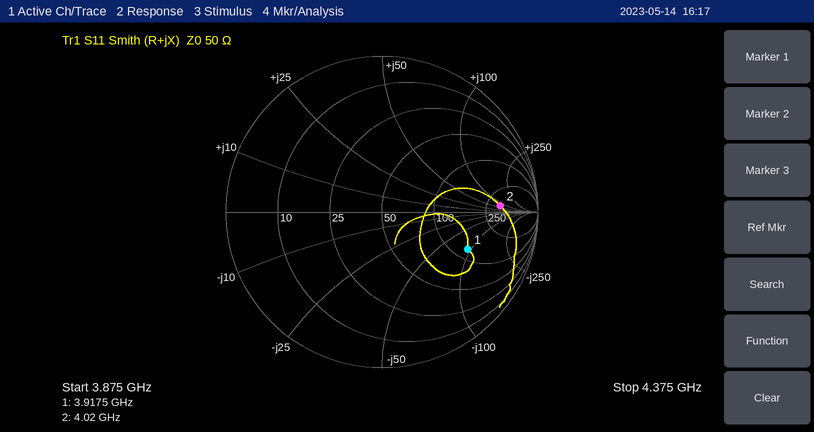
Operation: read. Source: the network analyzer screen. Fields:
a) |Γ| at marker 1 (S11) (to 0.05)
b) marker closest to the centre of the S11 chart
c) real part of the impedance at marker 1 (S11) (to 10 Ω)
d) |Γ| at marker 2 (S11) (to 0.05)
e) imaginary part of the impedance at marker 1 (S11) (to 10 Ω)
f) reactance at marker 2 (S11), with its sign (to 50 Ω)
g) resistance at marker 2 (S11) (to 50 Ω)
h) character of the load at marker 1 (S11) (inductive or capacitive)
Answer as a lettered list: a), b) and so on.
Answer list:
a) 0.60
b) marker 1
c) 120 Ω
d) 0.75
e) -90 Ω
f) +50 Ω
g) 350 Ω
h) capacitive
